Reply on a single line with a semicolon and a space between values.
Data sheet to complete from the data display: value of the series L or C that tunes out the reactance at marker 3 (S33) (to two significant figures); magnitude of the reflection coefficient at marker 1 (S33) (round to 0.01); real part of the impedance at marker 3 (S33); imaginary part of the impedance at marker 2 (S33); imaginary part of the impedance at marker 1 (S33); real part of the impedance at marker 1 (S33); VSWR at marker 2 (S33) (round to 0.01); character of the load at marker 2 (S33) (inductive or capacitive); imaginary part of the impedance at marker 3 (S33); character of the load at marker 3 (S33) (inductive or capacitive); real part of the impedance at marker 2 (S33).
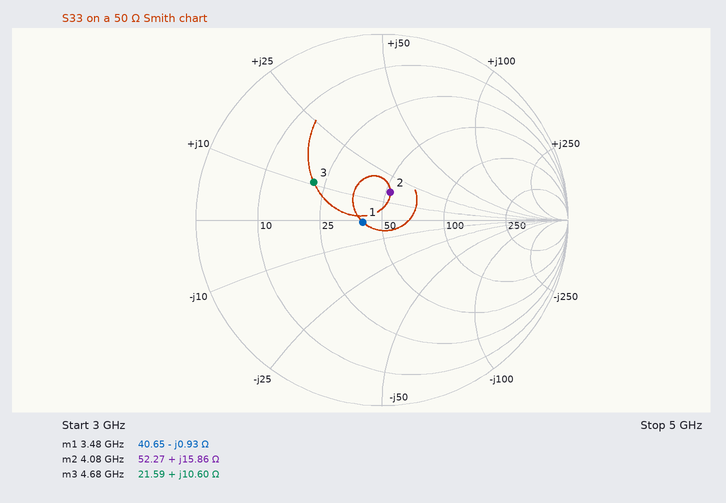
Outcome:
3.2 pF; 0.10; 21.59 Ω; +15.86 Ω; -0.93 Ω; 40.65 Ω; 1.37; inductive; +10.60 Ω; inductive; 52.27 Ω
